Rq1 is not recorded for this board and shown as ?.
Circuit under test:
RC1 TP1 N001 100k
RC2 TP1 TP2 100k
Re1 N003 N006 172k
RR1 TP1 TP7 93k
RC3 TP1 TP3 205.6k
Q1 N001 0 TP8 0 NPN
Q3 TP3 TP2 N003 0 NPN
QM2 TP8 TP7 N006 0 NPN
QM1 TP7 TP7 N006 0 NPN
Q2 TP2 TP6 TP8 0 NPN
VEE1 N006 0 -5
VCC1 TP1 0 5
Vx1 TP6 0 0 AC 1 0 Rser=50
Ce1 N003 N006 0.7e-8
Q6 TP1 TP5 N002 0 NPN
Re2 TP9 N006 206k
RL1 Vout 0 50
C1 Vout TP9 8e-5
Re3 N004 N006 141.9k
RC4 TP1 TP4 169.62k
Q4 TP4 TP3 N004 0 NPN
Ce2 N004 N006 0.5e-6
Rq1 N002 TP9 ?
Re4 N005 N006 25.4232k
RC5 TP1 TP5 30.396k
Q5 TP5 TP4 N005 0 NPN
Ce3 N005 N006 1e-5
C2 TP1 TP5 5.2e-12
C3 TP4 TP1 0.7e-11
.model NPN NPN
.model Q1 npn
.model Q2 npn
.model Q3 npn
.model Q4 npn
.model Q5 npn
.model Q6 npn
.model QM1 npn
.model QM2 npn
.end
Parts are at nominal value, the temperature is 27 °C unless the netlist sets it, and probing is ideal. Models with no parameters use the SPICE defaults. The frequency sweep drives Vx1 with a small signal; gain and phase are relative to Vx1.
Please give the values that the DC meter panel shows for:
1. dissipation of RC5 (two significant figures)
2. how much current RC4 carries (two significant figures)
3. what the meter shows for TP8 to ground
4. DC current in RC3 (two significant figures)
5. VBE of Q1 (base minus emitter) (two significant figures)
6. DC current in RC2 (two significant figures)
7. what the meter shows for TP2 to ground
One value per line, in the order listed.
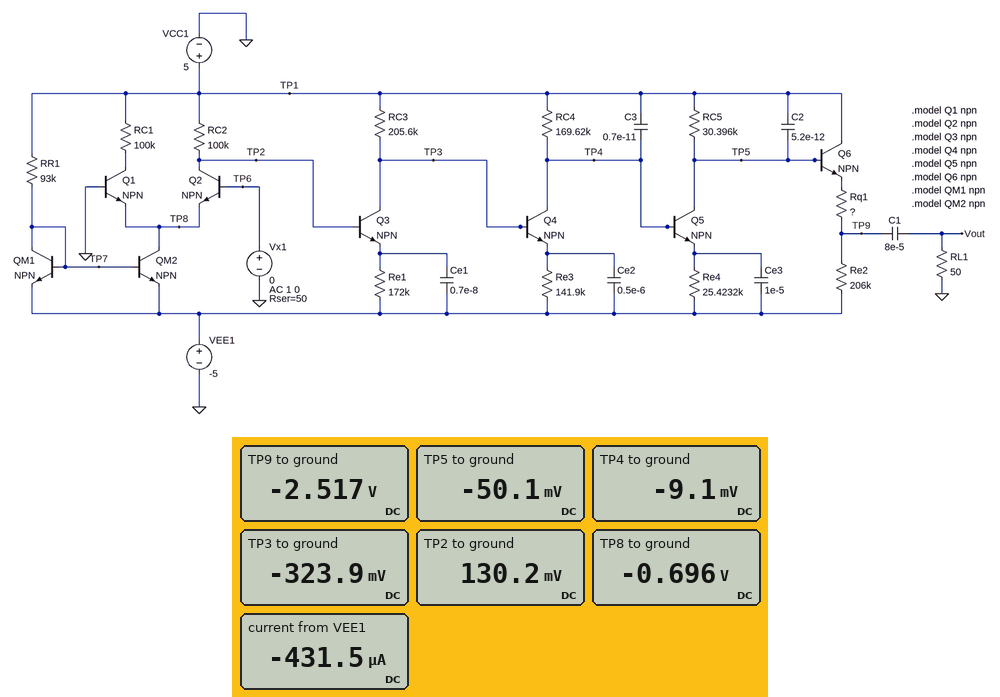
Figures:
840 µW
30 µA
-0.696 V
26 µA
700 mV
49 µA
130.2 mV
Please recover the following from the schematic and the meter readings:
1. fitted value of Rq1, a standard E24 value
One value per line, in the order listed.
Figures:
150 kΩ
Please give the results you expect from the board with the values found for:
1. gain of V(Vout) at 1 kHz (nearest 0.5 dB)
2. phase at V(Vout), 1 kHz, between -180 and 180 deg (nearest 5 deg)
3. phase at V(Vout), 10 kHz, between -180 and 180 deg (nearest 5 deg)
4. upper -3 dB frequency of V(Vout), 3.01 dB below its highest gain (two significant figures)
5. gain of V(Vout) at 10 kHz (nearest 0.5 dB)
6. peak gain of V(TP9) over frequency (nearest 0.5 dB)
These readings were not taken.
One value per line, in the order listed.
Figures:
47.5 dB
80 deg
35 deg
800 kHz
63.5 dB
65.5 dB
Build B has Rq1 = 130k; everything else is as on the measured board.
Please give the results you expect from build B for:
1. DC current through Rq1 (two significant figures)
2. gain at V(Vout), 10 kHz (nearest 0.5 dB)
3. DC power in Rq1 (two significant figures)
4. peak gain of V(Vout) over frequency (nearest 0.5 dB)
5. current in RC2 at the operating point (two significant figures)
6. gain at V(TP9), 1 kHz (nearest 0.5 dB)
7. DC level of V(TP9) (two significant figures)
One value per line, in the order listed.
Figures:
13 µA
64.5 dB
21 µW
66.5 dB
49 µA
49.0 dB
-2.4 V
